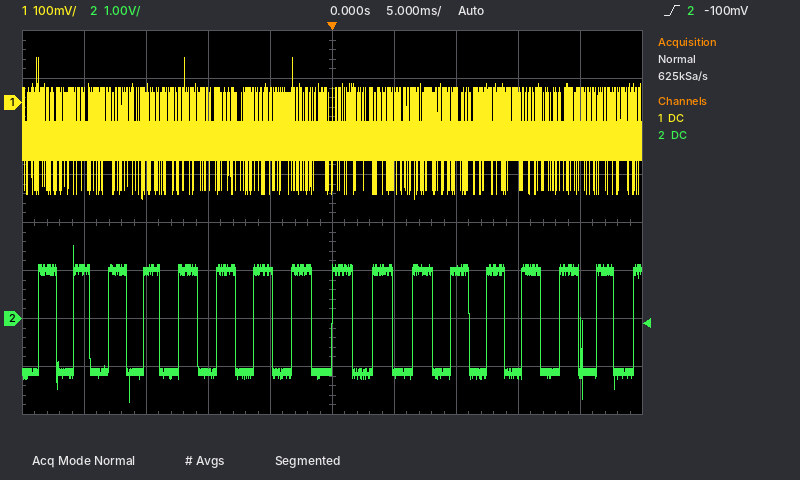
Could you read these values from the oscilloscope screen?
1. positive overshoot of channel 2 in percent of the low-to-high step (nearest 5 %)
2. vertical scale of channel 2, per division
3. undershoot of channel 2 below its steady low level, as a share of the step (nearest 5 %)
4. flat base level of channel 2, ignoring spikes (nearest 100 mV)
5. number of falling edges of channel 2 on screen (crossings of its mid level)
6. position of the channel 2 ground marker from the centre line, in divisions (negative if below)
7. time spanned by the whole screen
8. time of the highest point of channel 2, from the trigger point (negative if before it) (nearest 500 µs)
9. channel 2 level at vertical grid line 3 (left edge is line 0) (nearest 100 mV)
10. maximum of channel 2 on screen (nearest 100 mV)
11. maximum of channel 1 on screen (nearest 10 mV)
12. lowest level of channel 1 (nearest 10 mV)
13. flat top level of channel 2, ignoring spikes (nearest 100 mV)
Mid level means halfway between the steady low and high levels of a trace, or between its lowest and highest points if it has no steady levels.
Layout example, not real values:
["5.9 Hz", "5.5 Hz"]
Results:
["25 %", "1 V", "30 %", "-1.1 V", "16", "-2.0 div", "50 ms", "-21.0 ms", "-1.1 V", "1.5 V", "90 mV", "-200 mV", "1.0 V"]
